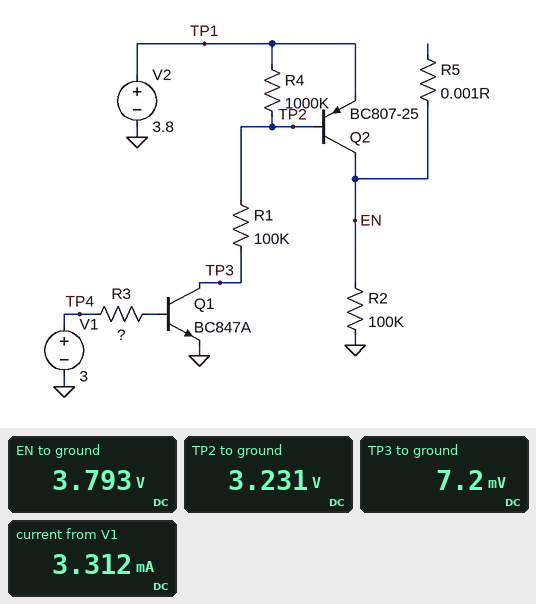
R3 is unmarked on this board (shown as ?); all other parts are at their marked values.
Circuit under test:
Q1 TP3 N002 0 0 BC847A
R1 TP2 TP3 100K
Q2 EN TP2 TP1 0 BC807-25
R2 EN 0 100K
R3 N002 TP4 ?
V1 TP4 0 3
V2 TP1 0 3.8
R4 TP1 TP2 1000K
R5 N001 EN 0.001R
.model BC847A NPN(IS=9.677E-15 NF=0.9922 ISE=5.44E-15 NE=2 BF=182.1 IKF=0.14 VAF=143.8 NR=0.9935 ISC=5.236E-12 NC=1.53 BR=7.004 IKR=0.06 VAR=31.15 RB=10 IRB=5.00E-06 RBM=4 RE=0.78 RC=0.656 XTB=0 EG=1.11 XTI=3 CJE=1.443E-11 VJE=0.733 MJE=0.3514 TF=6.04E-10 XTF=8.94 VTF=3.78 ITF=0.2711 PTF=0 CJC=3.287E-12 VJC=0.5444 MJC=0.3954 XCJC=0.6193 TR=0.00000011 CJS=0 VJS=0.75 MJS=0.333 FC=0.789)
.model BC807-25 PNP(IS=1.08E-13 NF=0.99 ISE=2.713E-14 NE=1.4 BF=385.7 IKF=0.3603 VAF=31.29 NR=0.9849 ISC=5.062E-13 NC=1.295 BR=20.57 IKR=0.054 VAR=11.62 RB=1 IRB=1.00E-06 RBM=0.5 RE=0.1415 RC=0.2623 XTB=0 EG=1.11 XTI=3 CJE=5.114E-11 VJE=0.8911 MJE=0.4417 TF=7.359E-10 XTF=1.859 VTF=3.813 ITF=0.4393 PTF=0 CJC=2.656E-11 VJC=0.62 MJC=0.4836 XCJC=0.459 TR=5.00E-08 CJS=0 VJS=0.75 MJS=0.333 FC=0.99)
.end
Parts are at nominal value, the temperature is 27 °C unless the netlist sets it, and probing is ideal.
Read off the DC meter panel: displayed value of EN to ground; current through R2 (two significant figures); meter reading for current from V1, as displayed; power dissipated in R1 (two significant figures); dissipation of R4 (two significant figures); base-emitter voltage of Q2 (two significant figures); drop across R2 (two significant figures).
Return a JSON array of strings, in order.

["3.793 V", "38 µA", "3.312 mA", "100 µW", "320 nW", "-570 mV", "3.8 V"]
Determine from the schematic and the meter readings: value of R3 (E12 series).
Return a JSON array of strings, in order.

["680 Ω"]
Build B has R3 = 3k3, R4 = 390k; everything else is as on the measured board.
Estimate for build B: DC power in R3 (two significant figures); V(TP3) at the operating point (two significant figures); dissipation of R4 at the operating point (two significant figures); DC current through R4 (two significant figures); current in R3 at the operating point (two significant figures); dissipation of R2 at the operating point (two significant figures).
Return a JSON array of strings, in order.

["1.6 mW", "4.8 mV", "830 nW", "1.5 µA", "700 µA", "140 µW"]
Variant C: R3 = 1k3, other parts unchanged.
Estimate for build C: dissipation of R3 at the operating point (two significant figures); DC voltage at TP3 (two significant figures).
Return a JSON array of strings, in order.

["4.0 mW", "5.6 mV"]
